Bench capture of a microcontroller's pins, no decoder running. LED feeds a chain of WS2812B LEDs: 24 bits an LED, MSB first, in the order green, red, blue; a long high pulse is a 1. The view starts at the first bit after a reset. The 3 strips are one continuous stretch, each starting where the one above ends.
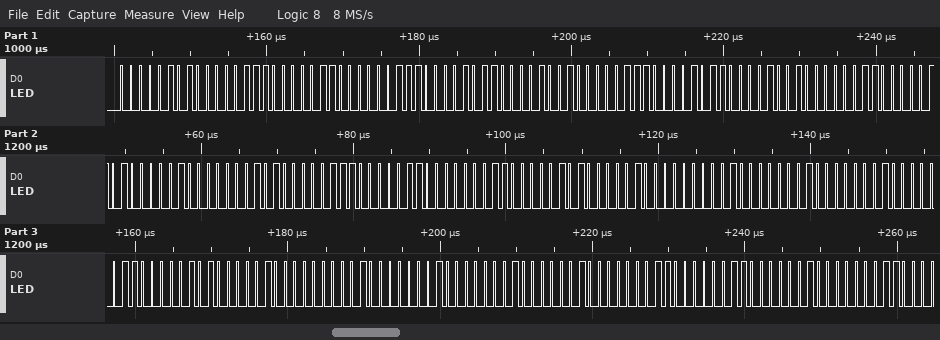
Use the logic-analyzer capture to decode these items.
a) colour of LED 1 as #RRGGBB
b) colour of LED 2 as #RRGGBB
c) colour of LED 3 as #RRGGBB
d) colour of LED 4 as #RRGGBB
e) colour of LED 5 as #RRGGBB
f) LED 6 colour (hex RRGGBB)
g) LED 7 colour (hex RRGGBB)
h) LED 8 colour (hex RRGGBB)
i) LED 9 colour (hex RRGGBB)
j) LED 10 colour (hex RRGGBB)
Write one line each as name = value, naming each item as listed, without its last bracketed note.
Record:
colour of LED 1 as #RRGGBB = #070506
colour of LED 2 as #RRGGBB = #0B0709
colour of LED 3 as #RRGGBB = #0B0709
colour of LED 4 as #RRGGBB = #050304
colour of LED 5 as #RRGGBB = #070506
LED 6 colour = #050304
LED 7 colour = #010101
LED 8 colour = #050304
LED 9 colour = #010101
LED 10 colour = #030203
